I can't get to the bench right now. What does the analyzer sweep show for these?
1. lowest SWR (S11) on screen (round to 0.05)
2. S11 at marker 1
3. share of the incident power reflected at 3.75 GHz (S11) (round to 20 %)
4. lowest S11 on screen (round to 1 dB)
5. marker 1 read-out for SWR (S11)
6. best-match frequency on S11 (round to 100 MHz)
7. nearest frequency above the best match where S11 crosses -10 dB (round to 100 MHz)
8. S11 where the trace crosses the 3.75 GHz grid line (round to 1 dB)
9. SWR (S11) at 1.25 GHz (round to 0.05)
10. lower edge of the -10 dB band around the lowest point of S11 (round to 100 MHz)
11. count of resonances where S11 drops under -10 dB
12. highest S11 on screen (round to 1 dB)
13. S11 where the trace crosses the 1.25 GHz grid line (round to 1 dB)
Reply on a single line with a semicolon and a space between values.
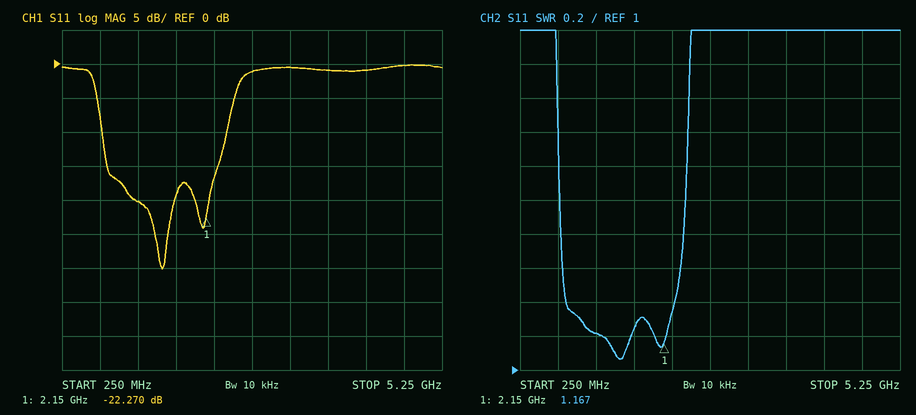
1.05; -22.270 dB; 80 %; -30 dB; 1.167; 1.6 GHz; 2.4 GHz; -1 dB; 1.20; 800 MHz; 2; 0 dB; -20 dB
